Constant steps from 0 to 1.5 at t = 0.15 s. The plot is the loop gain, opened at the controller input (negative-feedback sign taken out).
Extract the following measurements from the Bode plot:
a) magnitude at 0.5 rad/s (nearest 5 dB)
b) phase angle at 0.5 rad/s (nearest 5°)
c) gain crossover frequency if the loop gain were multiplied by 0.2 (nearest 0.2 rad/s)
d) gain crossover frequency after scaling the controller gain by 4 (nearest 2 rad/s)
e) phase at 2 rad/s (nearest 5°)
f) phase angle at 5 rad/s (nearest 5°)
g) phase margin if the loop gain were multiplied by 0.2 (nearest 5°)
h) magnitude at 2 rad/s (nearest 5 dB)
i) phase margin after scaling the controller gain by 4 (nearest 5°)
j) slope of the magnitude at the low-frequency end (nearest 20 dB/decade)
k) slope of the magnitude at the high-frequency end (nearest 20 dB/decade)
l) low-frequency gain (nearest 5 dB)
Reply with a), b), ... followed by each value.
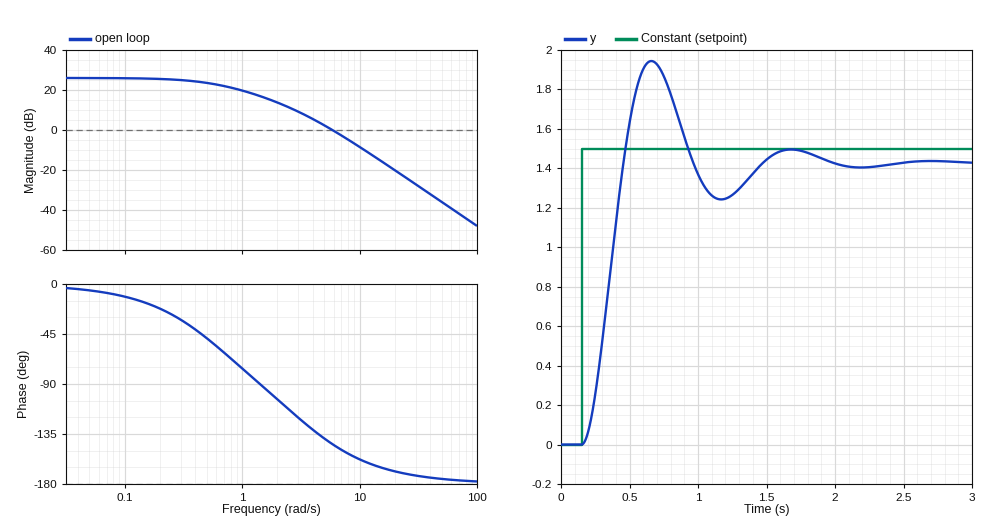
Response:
a) 25 dB
b) -50°
c) 2.0 rad/s
d) 12 rad/s
e) -105°
f) -140°
g) 75°
h) 15 dB
i) 20°
j) 0 dB/decade
k) -40 dB/decade
l) 25 dB
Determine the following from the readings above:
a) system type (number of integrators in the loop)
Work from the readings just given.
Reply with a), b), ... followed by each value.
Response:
a) 0
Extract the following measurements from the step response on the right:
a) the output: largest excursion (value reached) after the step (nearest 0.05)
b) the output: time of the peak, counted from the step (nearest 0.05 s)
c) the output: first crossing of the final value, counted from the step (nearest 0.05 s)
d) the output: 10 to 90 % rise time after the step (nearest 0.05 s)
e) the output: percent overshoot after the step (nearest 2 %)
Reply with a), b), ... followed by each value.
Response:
a) 1.95
b) 0.50 s
c) 0.30 s
d) 0.20 s
e) 36 %
